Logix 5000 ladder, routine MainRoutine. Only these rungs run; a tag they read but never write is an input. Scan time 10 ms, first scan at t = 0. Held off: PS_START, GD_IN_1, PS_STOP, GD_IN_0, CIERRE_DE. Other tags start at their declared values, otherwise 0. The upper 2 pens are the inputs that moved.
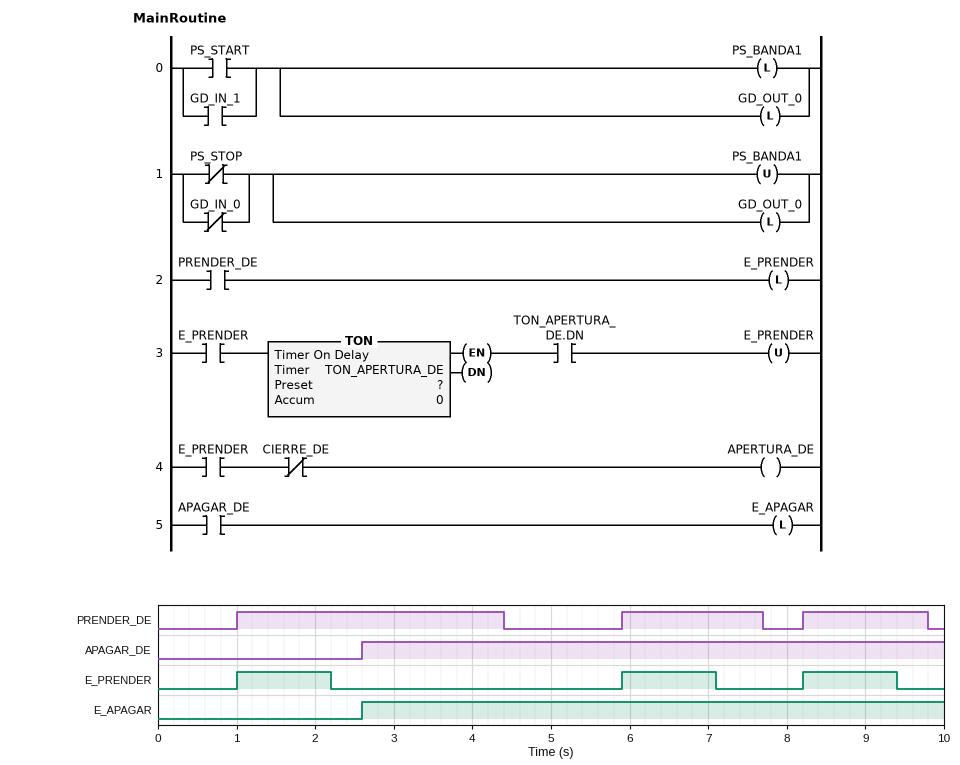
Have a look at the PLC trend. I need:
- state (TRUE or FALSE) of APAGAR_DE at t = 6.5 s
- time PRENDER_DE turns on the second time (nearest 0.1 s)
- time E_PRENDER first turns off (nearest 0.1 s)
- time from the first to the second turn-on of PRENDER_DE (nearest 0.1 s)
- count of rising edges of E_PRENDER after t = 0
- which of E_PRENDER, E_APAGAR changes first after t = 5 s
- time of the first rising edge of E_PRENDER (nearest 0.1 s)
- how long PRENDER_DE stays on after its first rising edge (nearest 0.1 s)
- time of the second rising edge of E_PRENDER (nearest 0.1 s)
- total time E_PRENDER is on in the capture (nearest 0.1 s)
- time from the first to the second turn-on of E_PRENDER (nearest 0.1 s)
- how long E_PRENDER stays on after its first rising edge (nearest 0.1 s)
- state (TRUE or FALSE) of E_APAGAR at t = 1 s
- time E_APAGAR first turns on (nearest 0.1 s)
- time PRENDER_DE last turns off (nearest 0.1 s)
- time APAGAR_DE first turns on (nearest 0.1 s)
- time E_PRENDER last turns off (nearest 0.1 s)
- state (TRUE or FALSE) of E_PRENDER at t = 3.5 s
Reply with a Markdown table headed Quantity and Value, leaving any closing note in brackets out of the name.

| Quantity | Value |
|---|---|
| state (TRUE or FALSE) of APAGAR_DE at t = 6.5 s | TRUE |
| time PRENDER_DE turns on the second time | 5.9 s |
| time E_PRENDER first turns off | 2.2 s |
| time from the first to the second turn-on of PRENDER_DE | 4.9 s |
| count of rising edges of E_PRENDER after t = 0 | 3 |
| which of E_PRENDER, E_APAGAR changes first after t = 5 s | E_PRENDER |
| time of the first rising edge of E_PRENDER | 1.0 s |
| how long PRENDER_DE stays on after its first rising edge | 3.4 s |
| time of the second rising edge of E_PRENDER | 5.9 s |
| total time E_PRENDER is on in the capture | 3.6 s |
| time from the first to the second turn-on of E_PRENDER | 4.9 s |
| how long E_PRENDER stays on after its first rising edge | 1.2 s |
| state (TRUE or FALSE) of E_APAGAR at t = 1 s | FALSE |
| time E_APAGAR first turns on | 2.6 s |
| time PRENDER_DE last turns off | 9.8 s |
| time APAGAR_DE first turns on | 2.6 s |
| time E_PRENDER last turns off | 9.4 s |
| state (TRUE or FALSE) of E_PRENDER at t = 3.5 s | FALSE |
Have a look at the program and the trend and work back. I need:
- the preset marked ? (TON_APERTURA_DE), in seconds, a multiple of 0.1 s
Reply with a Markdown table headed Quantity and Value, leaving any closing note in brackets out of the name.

| Quantity | Value |
|---|---|
| the preset marked ? (TON_APERTURA_DE), in seconds, a multiple of 0.1 s | 1.2 s |
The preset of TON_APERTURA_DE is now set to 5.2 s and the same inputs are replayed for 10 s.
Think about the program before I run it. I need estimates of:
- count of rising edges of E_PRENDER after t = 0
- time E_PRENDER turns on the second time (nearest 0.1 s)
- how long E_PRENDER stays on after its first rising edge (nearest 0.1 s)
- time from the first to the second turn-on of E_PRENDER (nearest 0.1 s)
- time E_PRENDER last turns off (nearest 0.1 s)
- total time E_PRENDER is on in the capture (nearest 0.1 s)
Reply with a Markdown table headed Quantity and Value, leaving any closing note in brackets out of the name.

| Quantity | Value |
|---|---|
| count of rising edges of E_PRENDER after t = 0 | 2 |
| time E_PRENDER turns on the second time | 8.2 s |
| how long E_PRENDER stays on after its first rising edge | 5.2 s |
| time from the first to the second turn-on of E_PRENDER | 7.2 s |
| time E_PRENDER last turns off | 6.2 s |
| total time E_PRENDER is on in the capture | 7.0 s |
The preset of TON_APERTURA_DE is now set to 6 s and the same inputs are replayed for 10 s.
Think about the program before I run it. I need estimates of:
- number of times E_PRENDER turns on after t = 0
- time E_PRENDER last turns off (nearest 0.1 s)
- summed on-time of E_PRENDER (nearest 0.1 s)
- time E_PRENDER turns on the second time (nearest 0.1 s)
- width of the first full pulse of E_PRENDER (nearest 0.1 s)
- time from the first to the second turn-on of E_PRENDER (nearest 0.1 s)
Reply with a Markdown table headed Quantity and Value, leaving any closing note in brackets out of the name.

| Quantity | Value |
|---|---|
| number of times E_PRENDER turns on after t = 0 | 2 |
| time E_PRENDER last turns off | 7.0 s |
| summed on-time of E_PRENDER | 7.8 s |
| time E_PRENDER turns on the second time | 8.2 s |
| width of the first full pulse of E_PRENDER | 6.0 s |
| time from the first to the second turn-on of E_PRENDER | 7.2 s |
